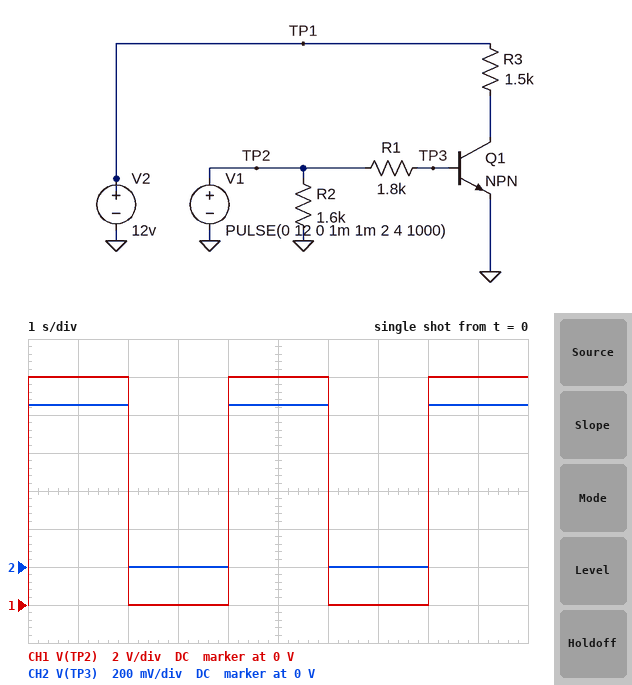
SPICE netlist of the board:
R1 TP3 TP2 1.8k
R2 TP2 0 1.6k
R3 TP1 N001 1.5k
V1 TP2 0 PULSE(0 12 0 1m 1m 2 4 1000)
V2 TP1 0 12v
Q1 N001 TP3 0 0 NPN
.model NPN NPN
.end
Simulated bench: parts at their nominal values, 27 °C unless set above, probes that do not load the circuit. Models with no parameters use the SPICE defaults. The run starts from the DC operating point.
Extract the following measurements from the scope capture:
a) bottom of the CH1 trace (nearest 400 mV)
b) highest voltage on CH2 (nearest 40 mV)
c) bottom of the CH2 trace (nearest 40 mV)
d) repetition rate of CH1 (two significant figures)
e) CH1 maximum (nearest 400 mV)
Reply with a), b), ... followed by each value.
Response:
a) 0 V
b) 840 mV
c) 0 V
d) 250 mHz
e) 12.0 V
